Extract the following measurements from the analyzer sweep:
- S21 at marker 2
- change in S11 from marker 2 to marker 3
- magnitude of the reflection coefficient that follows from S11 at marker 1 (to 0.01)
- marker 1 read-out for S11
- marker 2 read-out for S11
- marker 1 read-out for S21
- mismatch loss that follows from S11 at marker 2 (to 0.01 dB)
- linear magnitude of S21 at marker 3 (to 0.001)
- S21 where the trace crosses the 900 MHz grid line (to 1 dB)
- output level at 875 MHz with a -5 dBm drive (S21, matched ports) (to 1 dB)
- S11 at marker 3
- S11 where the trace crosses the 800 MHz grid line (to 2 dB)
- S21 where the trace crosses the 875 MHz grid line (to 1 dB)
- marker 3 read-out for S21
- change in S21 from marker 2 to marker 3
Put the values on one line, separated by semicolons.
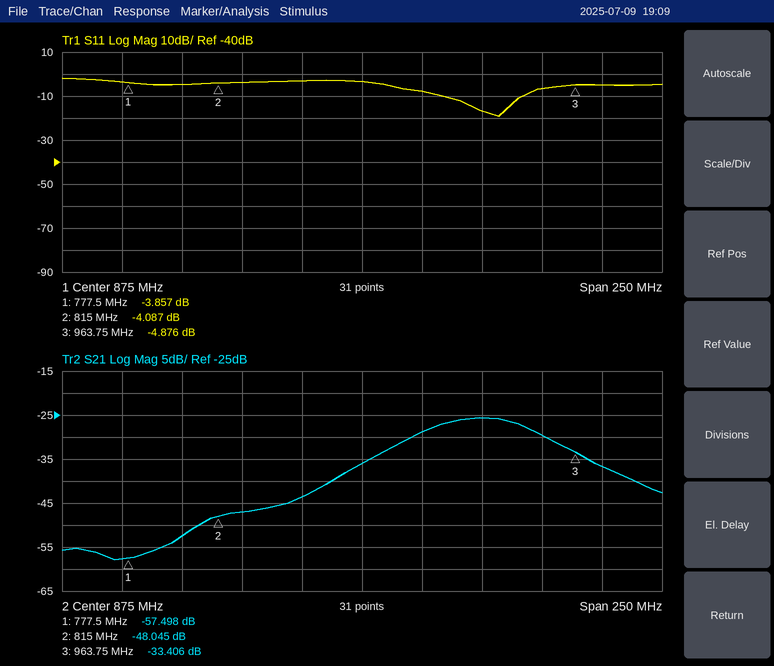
-48.045 dB; -0.789 dB; 0.64; -3.857 dB; -4.087 dB; -57.498 dB; 2.15 dB; 0.021; -29 dB; -41 dBm; -4.876 dB; -4 dB; -36 dB; -33.406 dB; 14.639 dB
